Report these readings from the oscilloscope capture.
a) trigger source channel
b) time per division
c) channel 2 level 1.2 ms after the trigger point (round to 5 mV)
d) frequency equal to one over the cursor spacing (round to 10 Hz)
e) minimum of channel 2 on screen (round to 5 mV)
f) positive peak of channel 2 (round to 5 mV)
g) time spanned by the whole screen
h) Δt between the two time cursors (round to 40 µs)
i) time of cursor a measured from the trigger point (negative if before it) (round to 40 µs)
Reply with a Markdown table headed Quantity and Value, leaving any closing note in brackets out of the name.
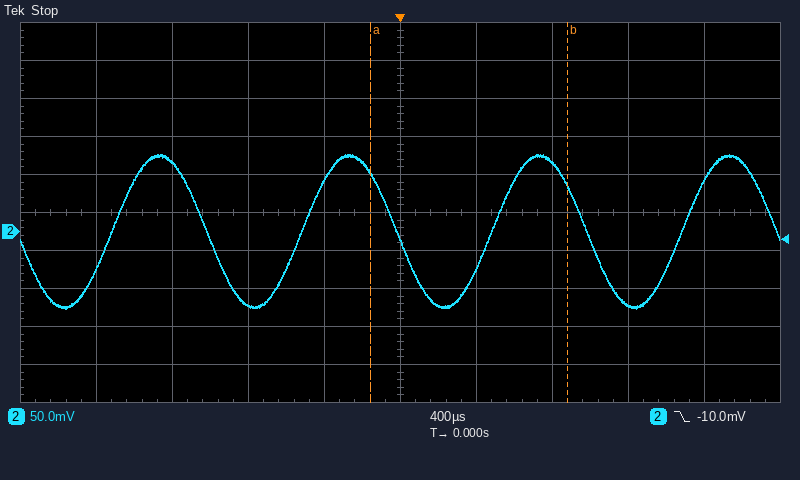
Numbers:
| Quantity | Value |
|---|---|
| trigger source channel | channel 2 |
| time per division | 400 µs |
| channel 2 level 1.2 ms after the trigger point | -95 mV |
| frequency equal to one over the cursor spacing | 960 Hz |
| minimum of channel 2 on screen | -100 mV |
| positive peak of channel 2 | 100 mV |
| time spanned by the whole screen | 4 ms |
| Δt between the two time cursors | 1.04 ms |
| time of cursor a measured from the trigger point (negative if before it) | -160 µs |
